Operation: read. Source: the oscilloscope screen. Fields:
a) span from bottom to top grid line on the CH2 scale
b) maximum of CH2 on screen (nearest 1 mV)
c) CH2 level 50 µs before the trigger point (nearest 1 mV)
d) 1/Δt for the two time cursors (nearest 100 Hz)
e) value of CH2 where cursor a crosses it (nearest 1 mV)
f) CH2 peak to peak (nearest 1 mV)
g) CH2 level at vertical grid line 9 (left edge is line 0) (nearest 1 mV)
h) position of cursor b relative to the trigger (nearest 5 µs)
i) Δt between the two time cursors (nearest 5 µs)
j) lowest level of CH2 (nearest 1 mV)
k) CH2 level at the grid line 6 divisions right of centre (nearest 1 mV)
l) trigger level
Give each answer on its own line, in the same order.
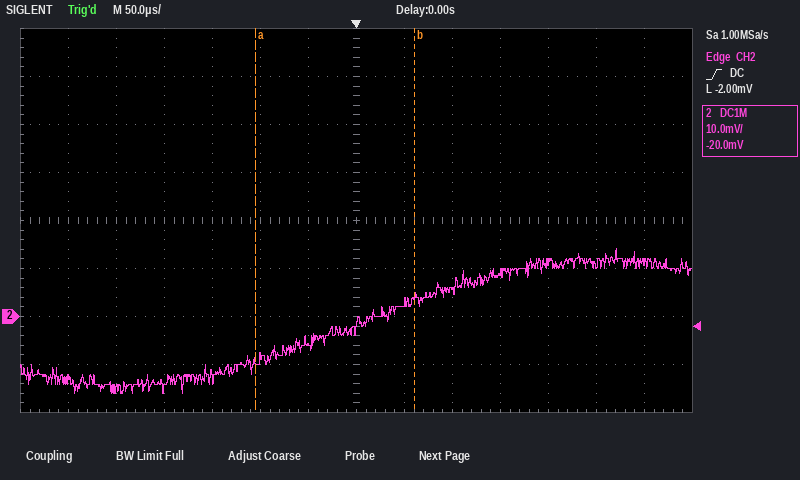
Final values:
80 mV
14 mV
-6 mV
6.1 kHz
-10 mV
30 mV
5 mV
+60 µs
165 µs
-16 mV
11 mV
-2.00 mV
